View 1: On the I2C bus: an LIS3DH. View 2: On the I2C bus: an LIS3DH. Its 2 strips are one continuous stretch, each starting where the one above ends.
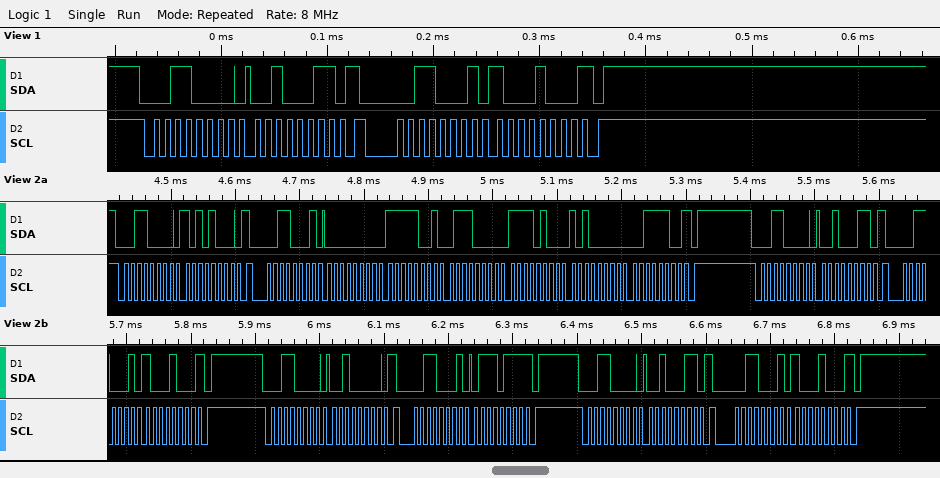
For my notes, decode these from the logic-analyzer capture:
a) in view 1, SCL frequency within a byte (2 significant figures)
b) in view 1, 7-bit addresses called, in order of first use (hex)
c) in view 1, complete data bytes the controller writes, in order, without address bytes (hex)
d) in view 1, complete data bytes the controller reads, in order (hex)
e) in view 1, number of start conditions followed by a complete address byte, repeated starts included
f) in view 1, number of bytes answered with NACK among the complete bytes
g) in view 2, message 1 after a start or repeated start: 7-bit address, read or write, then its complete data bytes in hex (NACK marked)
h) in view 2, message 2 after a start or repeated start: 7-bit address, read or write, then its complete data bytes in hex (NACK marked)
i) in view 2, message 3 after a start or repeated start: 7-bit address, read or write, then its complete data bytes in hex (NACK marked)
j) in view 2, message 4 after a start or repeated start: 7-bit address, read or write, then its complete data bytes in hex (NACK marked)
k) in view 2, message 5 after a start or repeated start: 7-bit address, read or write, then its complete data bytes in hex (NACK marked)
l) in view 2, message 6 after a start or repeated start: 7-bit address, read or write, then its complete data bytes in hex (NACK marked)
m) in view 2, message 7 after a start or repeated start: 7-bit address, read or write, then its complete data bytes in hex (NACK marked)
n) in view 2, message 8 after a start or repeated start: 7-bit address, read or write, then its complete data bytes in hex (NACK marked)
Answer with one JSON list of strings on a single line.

["100 kHz", "0x18", "23", "88", "2", "1", "0x18 write: A8", "0x18 read: 00 F9 70 F4 A0 3C NACK", "0x18 write: 23", "0x18 read: 88 NACK", "0x18 write: 20", "0x18 read: 77 NACK", "0x18 write: 23", "0x18 read: 88 NACK"]
